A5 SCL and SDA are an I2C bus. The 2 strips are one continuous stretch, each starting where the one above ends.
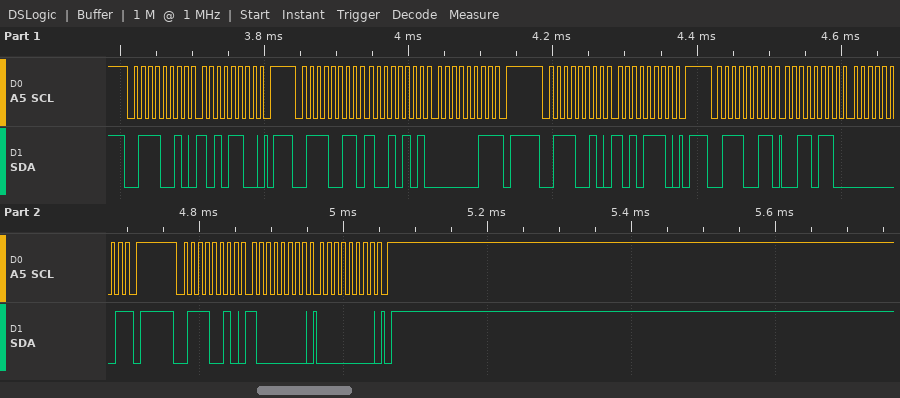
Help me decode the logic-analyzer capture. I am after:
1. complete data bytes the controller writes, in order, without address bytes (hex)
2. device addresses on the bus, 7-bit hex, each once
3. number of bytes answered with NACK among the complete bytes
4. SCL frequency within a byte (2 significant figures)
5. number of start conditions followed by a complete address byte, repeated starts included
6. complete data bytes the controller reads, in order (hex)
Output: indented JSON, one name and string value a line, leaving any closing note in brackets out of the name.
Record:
{
  "complete data bytes the controller writes, in order, without address bytes": "AC AE 80 00",
  "device addresses on the bus, 7-bit hex, each once": "0x39",
  "number of bytes answered with NACK among the complete bytes": "2",
  "SCL frequency within a byte": "100 kHz",
  "number of start conditions followed by a complete address byte, repeated starts included": "5",
  "complete data bytes the controller reads, in order": "95 03 36 01"
}
